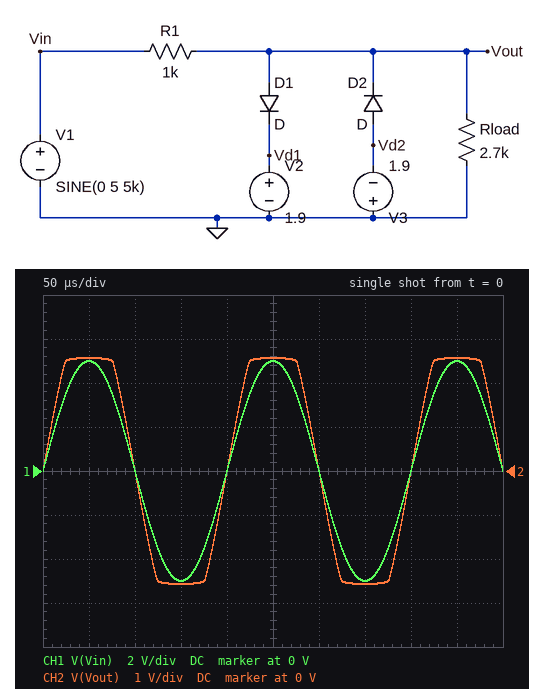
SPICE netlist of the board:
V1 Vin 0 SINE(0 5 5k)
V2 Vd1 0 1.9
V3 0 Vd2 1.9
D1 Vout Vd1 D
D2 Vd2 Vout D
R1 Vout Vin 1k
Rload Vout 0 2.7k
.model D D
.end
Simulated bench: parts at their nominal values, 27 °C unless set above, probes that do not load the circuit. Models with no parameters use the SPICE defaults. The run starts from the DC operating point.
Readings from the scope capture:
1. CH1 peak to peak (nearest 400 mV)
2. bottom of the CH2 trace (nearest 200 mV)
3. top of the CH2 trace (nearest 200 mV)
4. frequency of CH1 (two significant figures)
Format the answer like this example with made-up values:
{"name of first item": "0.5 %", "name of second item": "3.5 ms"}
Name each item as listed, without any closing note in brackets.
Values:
{"CH1 peak to peak": "10.0 V", "bottom of the CH2 trace": "-2.6 V", "top of the CH2 trace": "2.6 V", "frequency of CH1": "5.0 kHz"}
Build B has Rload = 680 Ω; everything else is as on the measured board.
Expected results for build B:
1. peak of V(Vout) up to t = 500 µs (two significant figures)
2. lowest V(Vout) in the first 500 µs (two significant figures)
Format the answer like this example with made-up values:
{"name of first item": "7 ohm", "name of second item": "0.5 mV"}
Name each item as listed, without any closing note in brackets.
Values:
{"peak of V(Vout) up to t = 500 µs": "2.0 V", "lowest V(Vout) in the first 500 µs": "-2.0 V"}
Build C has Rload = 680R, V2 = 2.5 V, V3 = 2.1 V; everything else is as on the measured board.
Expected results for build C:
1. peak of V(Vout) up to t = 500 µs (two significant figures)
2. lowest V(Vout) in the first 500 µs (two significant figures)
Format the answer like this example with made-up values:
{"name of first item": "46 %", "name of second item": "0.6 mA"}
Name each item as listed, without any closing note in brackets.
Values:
{"peak of V(Vout) up to t = 500 µs": "2.0 V", "lowest V(Vout) in the first 500 µs": "-2.0 V"}
